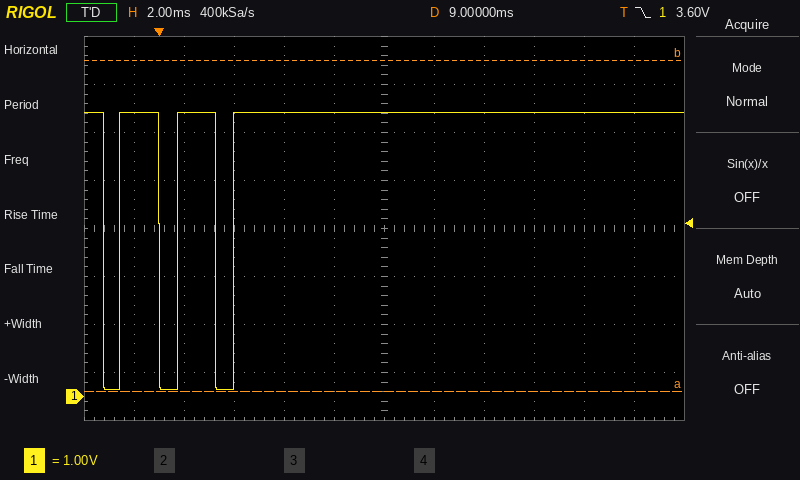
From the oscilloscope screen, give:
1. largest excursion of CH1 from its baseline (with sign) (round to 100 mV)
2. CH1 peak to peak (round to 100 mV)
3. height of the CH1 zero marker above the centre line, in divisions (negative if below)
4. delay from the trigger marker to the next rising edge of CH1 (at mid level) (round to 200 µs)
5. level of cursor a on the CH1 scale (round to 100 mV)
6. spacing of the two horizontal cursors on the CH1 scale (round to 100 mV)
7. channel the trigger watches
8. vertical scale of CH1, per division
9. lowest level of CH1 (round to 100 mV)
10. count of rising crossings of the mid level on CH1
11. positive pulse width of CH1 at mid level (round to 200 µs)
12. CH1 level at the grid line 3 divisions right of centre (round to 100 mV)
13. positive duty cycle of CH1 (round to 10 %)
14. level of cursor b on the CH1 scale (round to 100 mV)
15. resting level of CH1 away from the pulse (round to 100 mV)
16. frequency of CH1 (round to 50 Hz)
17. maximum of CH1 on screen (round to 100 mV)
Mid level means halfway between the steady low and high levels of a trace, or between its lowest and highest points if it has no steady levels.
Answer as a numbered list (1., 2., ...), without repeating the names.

1. -5.8 V
2. 5.8 V
3. -3.5 div
4. 800 µs
5. 100 mV
6. 6.9 V
7. CH1
8. 1 V
9. 100 mV
10. 3
11. 1.6 ms
12. 5.9 V
13. 70 %
14. 7.0 V
15. 5.9 V
16. 450 Hz
17. 5.9 V
